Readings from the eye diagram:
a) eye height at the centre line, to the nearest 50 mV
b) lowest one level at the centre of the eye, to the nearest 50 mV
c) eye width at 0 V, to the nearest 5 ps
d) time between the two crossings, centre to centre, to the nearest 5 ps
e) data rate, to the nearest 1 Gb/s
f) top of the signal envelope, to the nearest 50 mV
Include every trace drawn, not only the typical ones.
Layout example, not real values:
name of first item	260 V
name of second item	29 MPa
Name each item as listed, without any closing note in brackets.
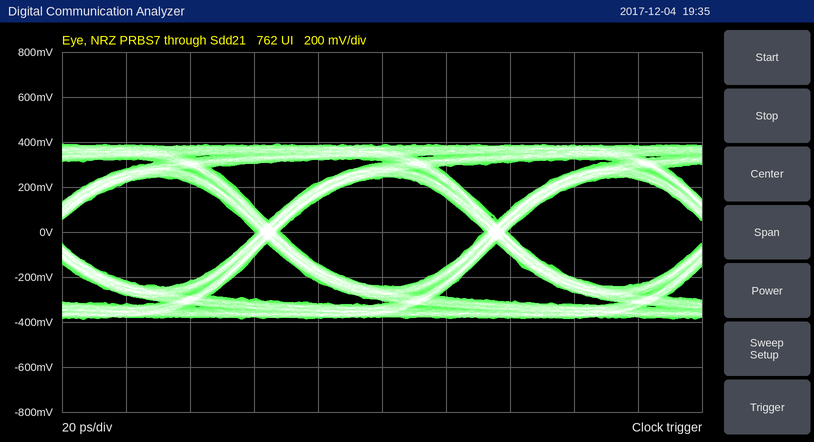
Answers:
eye height at the centre line, to the nearest 50 mV	500 mV
lowest one level at the centre of the eye, to the nearest 50 mV	250 mV
eye width at 0 V, to the nearest 5 ps	65 ps
time between the two crossings, centre to centre, to the nearest 5 ps	70 ps
data rate, to the nearest 1 Gb/s	14 Gb/s
top of the signal envelope, to the nearest 50 mV	400 mV
